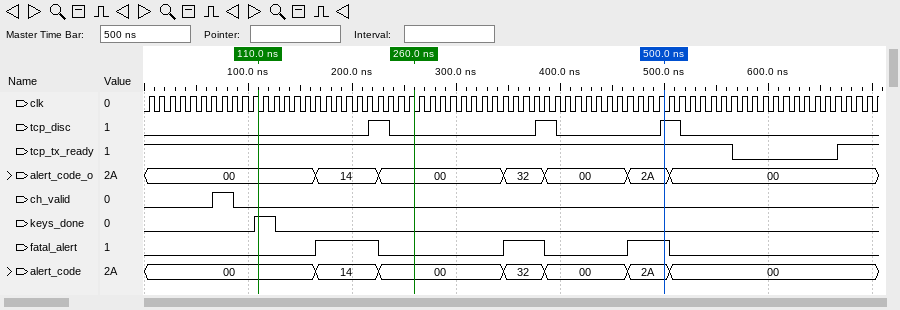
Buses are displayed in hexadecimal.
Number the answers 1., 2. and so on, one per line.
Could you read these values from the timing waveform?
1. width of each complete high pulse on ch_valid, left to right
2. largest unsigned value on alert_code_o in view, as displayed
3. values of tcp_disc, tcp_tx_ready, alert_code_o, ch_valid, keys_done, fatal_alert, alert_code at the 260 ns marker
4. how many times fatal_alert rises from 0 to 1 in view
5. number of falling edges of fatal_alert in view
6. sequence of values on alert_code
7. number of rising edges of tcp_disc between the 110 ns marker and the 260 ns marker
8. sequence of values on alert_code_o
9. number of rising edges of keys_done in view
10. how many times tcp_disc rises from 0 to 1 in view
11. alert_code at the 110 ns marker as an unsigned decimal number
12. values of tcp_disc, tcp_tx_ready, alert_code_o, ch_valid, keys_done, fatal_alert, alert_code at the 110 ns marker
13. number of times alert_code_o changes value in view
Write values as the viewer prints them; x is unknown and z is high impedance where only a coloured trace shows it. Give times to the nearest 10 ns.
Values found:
1. 20 ns
2. 32
3. tcp_disc=0, tcp_tx_ready=1, alert_code_o=00, ch_valid=0, keys_done=0, fatal_alert=0, alert_code=00
4. 3
5. 3
6. 00, 14, 00, 32, 00, 2A, 00
7. 1
8. 00, 14, 00, 32, 00, 2A, 00
9. 1
10. 3
11. 0
12. tcp_disc=0, tcp_tx_ready=1, alert_code_o=00, ch_valid=0, keys_done=1, fatal_alert=0, alert_code=00
13. 6
